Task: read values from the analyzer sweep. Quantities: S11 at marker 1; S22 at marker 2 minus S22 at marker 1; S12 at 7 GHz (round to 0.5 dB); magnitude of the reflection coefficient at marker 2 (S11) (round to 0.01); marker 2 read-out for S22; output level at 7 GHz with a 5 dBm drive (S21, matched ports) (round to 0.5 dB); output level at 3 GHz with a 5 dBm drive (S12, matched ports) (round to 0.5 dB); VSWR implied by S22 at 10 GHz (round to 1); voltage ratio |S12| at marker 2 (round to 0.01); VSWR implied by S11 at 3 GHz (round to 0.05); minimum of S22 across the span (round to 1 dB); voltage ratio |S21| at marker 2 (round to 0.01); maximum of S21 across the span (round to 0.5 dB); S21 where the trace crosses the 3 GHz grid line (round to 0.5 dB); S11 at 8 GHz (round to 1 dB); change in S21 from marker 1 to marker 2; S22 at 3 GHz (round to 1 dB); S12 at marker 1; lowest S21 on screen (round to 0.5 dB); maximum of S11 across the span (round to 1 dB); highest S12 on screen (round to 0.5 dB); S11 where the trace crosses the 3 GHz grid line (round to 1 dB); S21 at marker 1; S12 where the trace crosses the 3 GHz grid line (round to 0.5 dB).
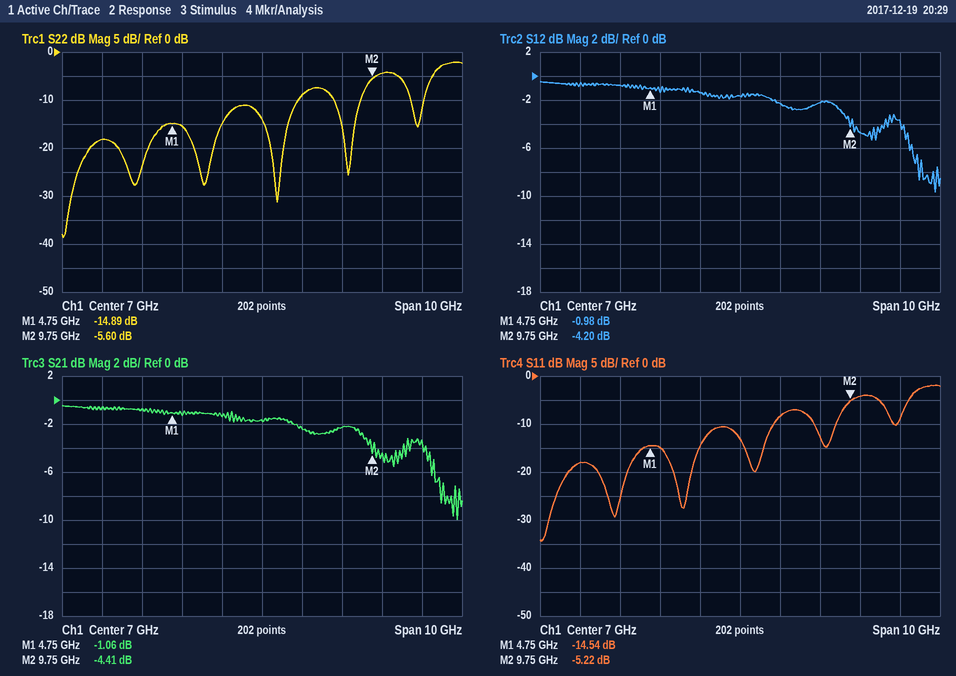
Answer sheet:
-14.54 dB
9.29 dB
-1.5 dB
0.55
-5.60 dB
3.5 dBm
4.5 dBm
4
0.62
1.30
-39 dB
0.60
-0.5 dB
-0.5 dB
-8 dB
-3.35 dB
-18 dB
-0.98 dB
-10.0 dB
-2 dB
-0.5 dB
-18 dB
-1.06 dB
-0.5 dB
